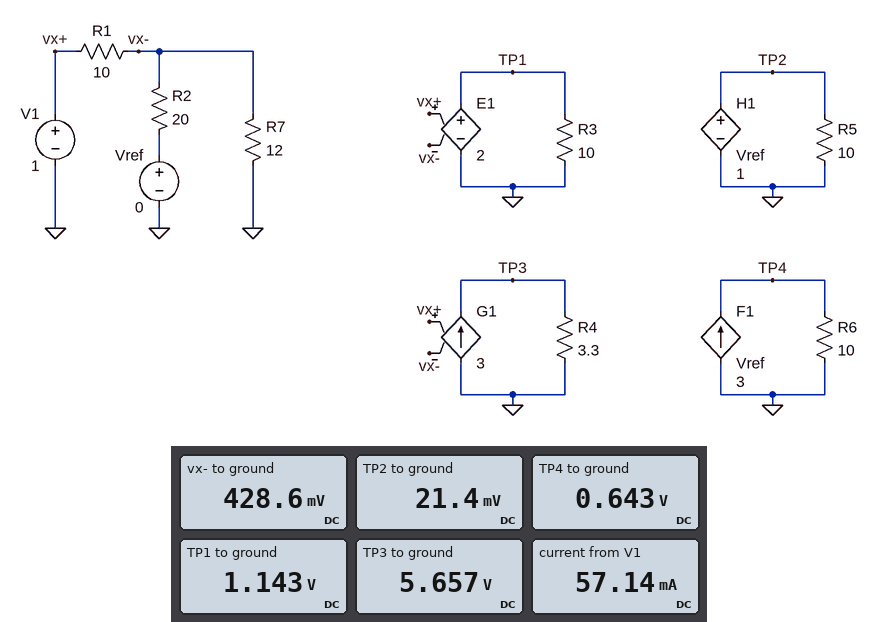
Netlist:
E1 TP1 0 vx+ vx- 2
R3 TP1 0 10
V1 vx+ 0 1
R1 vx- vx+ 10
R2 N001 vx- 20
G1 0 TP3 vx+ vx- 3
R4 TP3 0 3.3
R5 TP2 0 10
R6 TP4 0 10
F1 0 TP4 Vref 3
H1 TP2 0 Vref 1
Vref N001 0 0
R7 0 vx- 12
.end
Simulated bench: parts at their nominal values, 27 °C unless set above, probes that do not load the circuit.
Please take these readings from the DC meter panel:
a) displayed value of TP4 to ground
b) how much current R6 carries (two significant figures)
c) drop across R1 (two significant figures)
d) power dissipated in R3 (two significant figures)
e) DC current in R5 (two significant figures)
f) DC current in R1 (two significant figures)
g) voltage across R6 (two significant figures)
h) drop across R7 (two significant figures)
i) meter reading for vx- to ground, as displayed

0.643 V
64 mA
570 mV
130 mW
2.1 mA
57 mA
640 mV
430 mV
428.6 mV
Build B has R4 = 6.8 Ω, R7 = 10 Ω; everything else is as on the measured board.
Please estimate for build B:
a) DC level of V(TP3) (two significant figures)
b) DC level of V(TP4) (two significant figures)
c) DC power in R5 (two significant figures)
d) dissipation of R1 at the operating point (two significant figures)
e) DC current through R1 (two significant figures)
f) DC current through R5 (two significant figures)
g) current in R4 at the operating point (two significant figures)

12 V
600 mV
40 µW
36 mW
60 mA
2.0 mA
1.8 A
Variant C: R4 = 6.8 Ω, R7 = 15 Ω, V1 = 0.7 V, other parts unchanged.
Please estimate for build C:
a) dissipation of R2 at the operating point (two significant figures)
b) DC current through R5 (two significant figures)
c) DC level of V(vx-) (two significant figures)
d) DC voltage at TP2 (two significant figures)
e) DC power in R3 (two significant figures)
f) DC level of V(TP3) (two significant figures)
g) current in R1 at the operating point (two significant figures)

5.2 mW
1.6 mA
320 mV
16 mV
57 mW
7.7 V
38 mA
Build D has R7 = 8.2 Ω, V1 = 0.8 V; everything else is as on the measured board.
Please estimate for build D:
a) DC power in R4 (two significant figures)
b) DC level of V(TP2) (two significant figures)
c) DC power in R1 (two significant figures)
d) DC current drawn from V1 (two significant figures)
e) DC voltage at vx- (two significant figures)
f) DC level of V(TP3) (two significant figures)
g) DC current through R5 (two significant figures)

7.6 W
15 mV
26 mW
51 mA
290 mV
5.0 V
1.5 mA
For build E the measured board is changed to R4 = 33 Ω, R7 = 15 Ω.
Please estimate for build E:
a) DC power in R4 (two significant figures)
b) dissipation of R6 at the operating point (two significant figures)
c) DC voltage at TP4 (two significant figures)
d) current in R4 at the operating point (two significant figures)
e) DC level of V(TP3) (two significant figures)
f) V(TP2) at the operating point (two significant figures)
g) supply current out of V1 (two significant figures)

86 W
48 mW
690 mV
1.6 A
53 V
23 mV
54 mA
